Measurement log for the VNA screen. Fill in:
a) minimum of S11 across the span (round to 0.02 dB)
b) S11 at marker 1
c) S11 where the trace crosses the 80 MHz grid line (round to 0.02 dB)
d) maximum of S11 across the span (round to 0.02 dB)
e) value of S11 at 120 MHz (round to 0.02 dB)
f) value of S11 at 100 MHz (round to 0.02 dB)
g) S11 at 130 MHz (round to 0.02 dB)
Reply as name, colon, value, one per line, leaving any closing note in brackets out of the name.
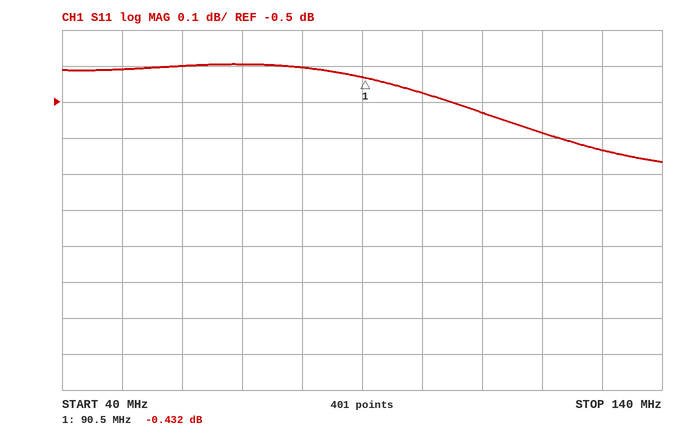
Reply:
minimum of S11 across the span: -0.66 dB
S11 at marker 1: -0.432 dB
S11 where the trace crosses the 80 MHz grid line: -0.40 dB
maximum of S11 across the span: -0.40 dB
value of S11 at 120 MHz: -0.58 dB
value of S11 at 100 MHz: -0.48 dB
S11 at 130 MHz: -0.64 dB
